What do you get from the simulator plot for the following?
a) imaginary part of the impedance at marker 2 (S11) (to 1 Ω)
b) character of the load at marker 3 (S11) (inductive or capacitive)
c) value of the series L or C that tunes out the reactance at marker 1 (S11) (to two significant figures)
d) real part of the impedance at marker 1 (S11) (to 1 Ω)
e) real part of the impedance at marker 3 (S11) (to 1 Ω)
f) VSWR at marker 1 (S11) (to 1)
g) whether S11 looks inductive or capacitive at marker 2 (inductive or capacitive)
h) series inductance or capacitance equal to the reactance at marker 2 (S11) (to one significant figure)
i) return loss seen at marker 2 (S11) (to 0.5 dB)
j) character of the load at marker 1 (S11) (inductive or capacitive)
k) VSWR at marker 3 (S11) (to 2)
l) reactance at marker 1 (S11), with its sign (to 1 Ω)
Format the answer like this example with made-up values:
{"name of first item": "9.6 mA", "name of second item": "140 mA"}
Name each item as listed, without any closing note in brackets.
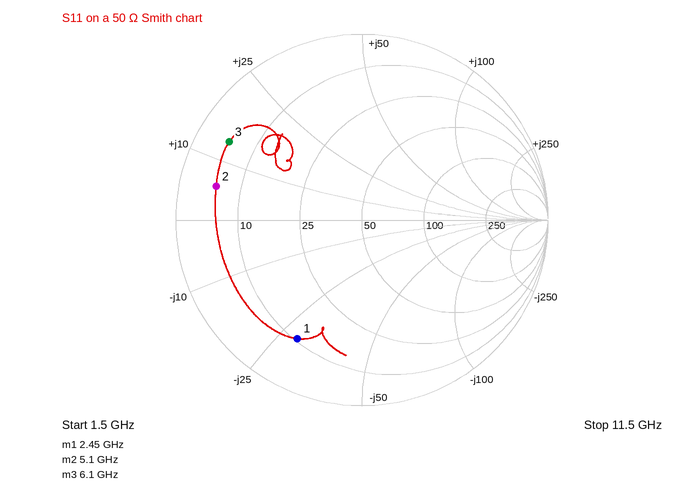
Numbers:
{"imaginary part of the impedance at marker 2 (S11)": "+6 Ω", "character of the load at marker 3 (S11)": "inductive", "value of the series L or C that tunes out the reactance at marker 1 (S11)": "1.9 nH", "real part of the impedance at marker 1 (S11)": "11 Ω", "real part of the impedance at marker 3 (S11)": "5 Ω", "VSWR at marker 1 (S11)": "6", "whether S11 looks inductive or capacitive at marker 2": "inductive", "series inductance or capacitance equal to the reactance at marker 2 (S11)": "200 pH", "return loss seen at marker 2 (S11)": "2.0 dB", "character of the load at marker 1 (S11)": "capacitive", "VSWR at marker 3 (S11)": "10", "reactance at marker 1 (S11), with its sign": "-29 Ω"}
